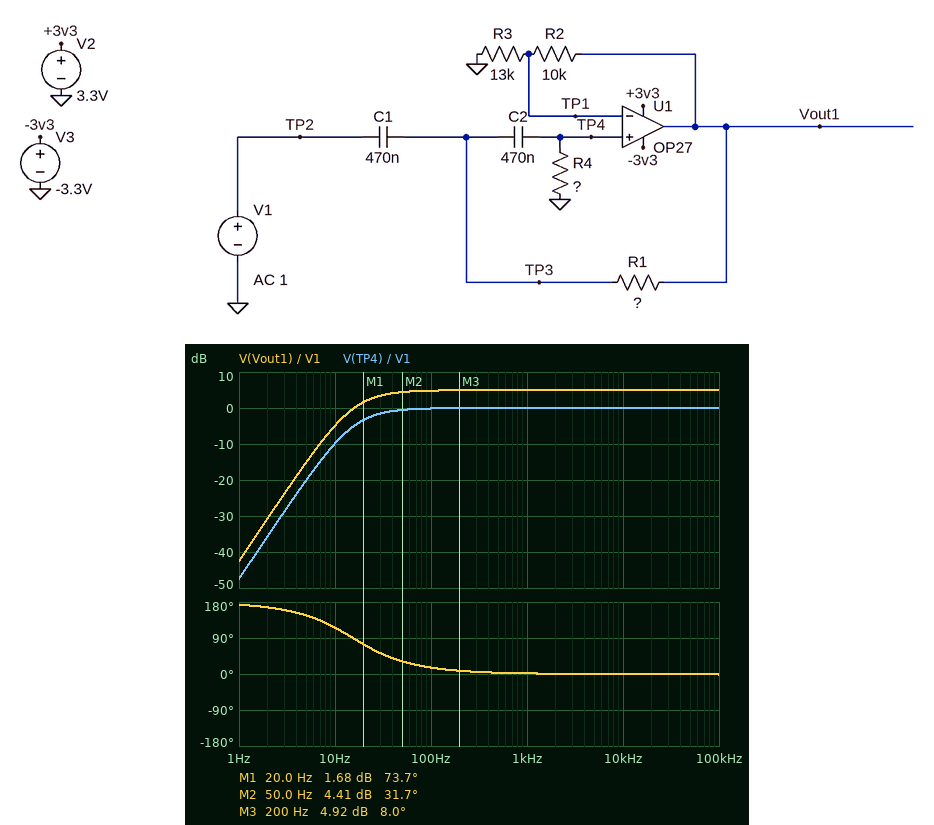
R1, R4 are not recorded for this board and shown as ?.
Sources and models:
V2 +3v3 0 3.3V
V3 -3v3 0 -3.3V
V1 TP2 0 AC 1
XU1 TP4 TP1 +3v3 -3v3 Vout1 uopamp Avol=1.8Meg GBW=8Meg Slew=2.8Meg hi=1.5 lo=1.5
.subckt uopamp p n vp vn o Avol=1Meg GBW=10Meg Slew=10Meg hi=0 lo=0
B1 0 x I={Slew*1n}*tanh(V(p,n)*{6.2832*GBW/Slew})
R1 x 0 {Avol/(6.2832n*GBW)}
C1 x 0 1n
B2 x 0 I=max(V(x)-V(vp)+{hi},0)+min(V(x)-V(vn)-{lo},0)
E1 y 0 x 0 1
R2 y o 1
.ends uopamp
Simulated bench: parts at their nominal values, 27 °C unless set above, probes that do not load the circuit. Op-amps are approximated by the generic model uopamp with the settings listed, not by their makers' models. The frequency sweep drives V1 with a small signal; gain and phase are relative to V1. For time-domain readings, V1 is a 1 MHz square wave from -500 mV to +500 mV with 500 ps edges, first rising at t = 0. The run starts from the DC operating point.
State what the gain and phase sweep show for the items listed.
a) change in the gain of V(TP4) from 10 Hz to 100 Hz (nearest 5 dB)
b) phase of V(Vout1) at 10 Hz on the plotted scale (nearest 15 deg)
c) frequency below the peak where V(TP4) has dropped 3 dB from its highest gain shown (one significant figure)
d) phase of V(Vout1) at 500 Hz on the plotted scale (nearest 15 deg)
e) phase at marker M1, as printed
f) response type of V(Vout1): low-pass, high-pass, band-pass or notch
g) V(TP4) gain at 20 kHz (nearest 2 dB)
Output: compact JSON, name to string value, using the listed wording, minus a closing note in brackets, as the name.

{"change in the gain of V(TP4) from 10 Hz to 100 Hz": "10 dB", "phase of V(Vout1) at 10 Hz on the plotted scale": "120 deg", "frequency below the peak where V(TP4) has dropped 3 dB from its highest gain shown": "20 Hz", "phase of V(Vout1) at 500 Hz on the plotted scale": "0 deg", "phase at marker M1, as printed": "73.7 deg", "response type of V(Vout1): low-pass, high-pass, band-pass or notch": "high-pass", "V(TP4) gain at 20 kHz": "0 dB"}
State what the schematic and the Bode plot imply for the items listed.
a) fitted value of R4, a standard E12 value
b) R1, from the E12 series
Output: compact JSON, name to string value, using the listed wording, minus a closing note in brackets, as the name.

{"fitted value of R4, a standard E12 value": "18 kΩ", "R1, from the E12 series": "27 kΩ"}
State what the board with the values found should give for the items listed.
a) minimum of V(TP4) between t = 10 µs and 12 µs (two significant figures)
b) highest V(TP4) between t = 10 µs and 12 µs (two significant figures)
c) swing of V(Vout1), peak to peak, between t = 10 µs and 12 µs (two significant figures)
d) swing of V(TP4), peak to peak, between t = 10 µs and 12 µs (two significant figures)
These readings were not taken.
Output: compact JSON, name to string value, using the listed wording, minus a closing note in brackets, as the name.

{"minimum of V(TP4) between t = 10 µs and 12 µs": "-1.2 mV", "highest V(TP4) between t = 10 µs and 12 µs": "1.0 V", "swing of V(Vout1), peak to peak, between t = 10 µs and 12 µs": "1.4 V", "swing of V(TP4), peak to peak, between t = 10 µs and 12 µs": "1.0 V"}
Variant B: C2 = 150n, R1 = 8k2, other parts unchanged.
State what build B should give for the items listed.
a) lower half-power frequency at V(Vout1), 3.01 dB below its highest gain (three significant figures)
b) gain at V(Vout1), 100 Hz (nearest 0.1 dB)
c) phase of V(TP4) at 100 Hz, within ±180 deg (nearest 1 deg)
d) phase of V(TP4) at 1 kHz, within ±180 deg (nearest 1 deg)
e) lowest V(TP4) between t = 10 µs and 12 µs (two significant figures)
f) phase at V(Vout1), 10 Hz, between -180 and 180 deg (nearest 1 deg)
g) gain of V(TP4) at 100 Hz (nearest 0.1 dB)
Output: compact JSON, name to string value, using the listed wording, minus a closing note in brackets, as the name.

{"lower half-power frequency at V(Vout1), 3.01 dB below its highest gain": "41.8 Hz", "gain at V(Vout1), 100 Hz": "6.0 dB", "phase of V(TP4) at 100 Hz, within ±180 deg": "31 deg", "phase of V(TP4) at 1 kHz, within ±180 deg": "3 deg", "lowest V(TP4) between t = 10 µs and 12 µs": "-2.1 mV", "phase at V(Vout1), 10 Hz, between -180 and 180 deg": "169 deg", "gain of V(TP4) at 100 Hz": "1.1 dB"}
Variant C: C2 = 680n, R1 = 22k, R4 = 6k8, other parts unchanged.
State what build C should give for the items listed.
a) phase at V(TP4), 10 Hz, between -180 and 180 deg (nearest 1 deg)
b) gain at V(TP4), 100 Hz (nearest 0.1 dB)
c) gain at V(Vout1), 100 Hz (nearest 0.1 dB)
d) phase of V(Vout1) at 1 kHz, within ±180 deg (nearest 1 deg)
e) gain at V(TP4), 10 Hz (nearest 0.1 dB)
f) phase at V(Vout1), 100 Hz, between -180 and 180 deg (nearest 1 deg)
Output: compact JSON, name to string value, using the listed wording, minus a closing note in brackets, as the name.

{"phase at V(TP4), 10 Hz, between -180 and 180 deg": "121 deg", "gain at V(TP4), 100 Hz": "-1.5 dB", "gain at V(Vout1), 100 Hz": "3.4 dB", "phase of V(Vout1) at 1 kHz, within ±180 deg": "4 deg", "gain at V(TP4), 10 Hz": "-18.5 dB", "phase at V(Vout1), 100 Hz, between -180 and 180 deg": "37 deg"}
